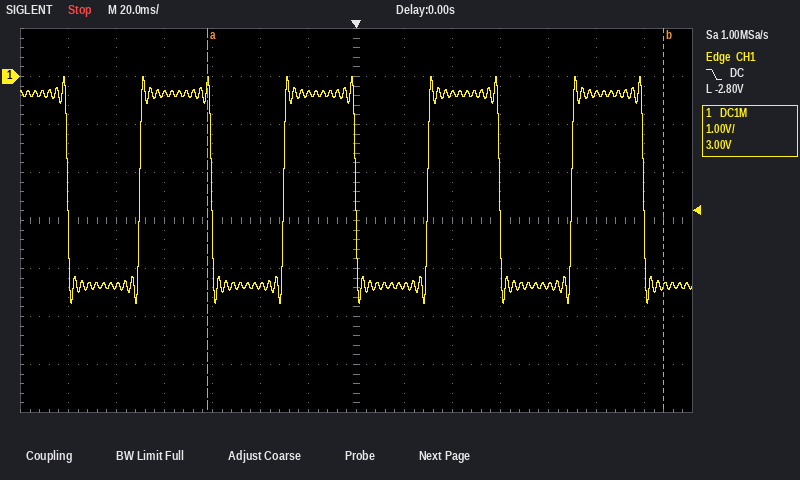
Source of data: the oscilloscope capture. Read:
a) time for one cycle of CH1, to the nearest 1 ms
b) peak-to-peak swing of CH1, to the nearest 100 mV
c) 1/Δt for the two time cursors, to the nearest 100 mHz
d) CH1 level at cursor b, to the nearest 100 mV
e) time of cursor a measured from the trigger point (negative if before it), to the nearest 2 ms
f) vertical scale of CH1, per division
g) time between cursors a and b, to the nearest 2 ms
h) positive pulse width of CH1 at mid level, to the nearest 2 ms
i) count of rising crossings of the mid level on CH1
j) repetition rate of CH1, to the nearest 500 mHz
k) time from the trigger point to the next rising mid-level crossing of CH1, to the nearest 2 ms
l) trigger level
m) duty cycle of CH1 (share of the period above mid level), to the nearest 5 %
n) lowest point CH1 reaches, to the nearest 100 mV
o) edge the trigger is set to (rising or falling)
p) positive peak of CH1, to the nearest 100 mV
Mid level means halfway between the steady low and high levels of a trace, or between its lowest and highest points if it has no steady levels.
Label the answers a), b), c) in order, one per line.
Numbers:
a) 60 ms
b) 4.7 V
c) 5.3 Hz
d) -4.4 V
e) -62 ms
f) 1 V
g) 190 ms
h) 30 ms
i) 4
j) 16.5 Hz
k) 30 ms
l) -2.80 V
m) 50 %
n) -4.7 V
o) falling
p) 0.0 V
